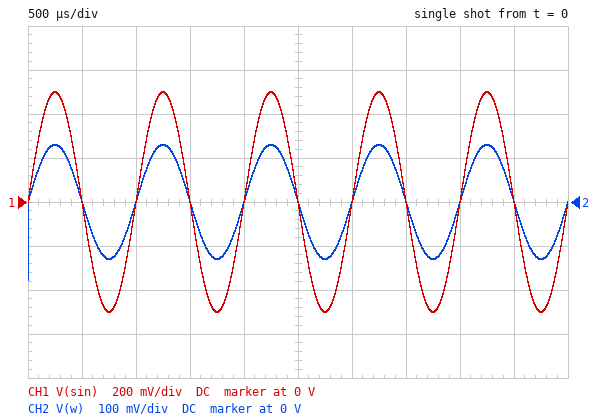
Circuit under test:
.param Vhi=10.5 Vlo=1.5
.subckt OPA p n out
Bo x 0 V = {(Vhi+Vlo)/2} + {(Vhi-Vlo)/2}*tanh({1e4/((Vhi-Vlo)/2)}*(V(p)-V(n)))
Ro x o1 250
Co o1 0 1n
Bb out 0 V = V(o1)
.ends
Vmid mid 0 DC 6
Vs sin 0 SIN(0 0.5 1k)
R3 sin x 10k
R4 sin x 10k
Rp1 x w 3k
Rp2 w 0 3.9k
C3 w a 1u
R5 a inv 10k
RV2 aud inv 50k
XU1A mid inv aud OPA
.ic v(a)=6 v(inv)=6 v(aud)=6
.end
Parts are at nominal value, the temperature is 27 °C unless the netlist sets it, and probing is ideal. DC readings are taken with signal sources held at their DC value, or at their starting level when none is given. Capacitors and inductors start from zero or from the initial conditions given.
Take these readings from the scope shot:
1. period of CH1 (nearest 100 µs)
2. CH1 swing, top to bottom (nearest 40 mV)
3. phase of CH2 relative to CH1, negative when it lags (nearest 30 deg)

1.0 ms
1.00 V
0 deg
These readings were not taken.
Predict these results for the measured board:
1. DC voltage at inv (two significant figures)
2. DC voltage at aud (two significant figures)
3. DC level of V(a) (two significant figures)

6.0 V
6.0 V
6.0 V
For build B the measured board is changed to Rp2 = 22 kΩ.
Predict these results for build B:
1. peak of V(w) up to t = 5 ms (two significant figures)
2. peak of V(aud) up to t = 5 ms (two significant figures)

230 mV
7.2 V
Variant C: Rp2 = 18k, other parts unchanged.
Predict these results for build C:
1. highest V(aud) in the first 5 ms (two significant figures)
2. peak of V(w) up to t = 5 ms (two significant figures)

7.1 V
220 mV
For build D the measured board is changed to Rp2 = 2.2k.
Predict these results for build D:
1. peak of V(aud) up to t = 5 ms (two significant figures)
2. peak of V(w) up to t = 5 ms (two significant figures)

6.5 V
92 mV
